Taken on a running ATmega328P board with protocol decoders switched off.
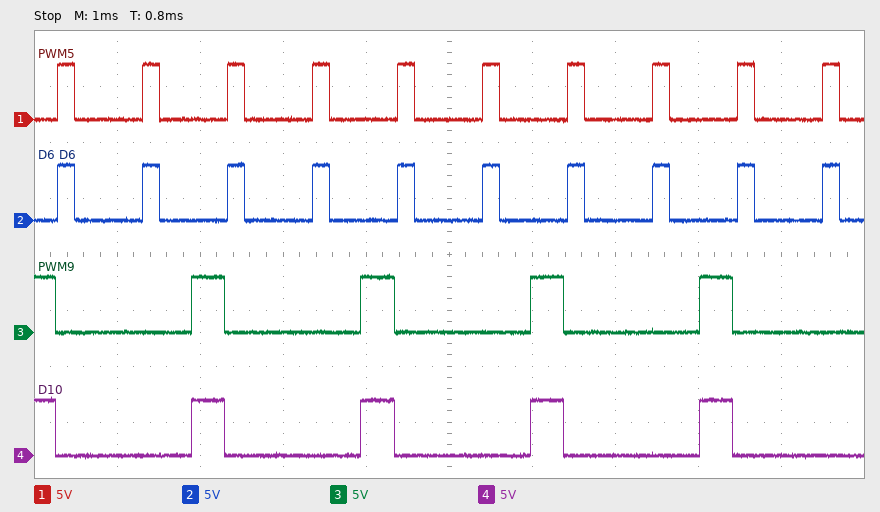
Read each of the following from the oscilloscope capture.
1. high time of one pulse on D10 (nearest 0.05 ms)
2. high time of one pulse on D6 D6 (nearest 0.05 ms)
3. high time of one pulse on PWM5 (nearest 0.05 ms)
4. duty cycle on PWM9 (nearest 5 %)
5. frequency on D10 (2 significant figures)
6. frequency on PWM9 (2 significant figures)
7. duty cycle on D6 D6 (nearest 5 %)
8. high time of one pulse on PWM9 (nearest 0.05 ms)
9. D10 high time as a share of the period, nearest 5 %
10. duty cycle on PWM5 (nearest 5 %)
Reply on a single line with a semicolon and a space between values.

0.40 ms; 0.20 ms; 0.20 ms; 20 %; 490 Hz; 490 Hz; 20 %; 0.40 ms; 20 %; 20 %
